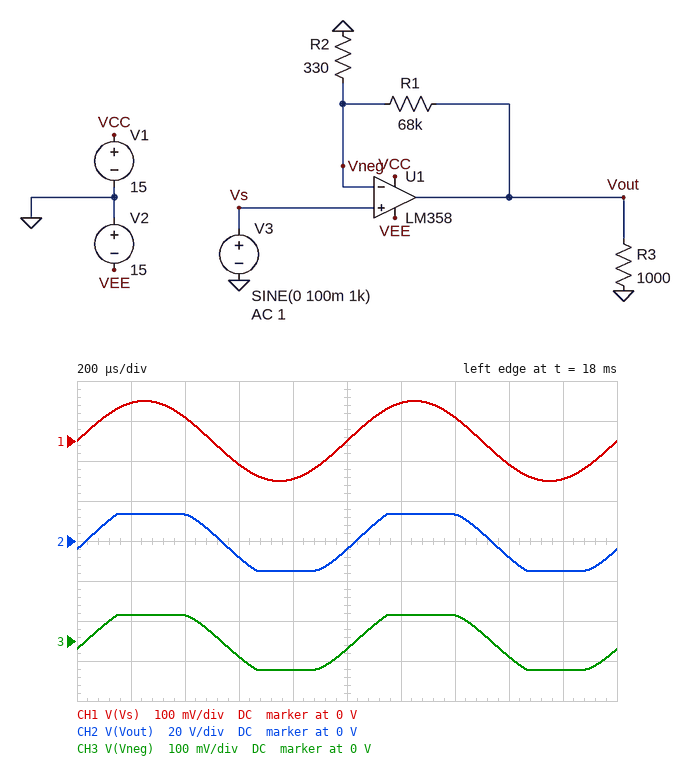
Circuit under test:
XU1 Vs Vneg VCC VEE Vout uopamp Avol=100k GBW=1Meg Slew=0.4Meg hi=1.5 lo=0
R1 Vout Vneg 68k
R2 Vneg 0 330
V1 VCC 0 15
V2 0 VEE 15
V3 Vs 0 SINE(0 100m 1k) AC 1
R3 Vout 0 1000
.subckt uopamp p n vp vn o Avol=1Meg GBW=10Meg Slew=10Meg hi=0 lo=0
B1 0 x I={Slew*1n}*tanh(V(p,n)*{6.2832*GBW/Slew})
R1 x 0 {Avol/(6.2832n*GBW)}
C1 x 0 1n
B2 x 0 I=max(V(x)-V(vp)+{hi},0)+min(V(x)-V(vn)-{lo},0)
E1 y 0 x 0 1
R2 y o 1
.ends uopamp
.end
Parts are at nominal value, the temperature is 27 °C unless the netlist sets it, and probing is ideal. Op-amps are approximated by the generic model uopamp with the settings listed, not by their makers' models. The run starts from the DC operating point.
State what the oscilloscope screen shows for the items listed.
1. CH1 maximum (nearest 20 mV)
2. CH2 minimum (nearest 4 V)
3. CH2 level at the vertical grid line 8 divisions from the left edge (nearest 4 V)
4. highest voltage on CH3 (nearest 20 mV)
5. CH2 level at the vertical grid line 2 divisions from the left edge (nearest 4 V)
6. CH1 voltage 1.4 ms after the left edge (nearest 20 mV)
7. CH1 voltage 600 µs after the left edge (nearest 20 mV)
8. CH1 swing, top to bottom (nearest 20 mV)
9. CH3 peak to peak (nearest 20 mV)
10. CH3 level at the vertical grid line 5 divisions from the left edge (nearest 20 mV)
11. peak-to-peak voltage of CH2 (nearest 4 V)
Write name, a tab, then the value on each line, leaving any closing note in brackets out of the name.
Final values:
CH1 maximum	100 mV
CH2 minimum	-16 V
CH2 level at the vertical grid line 8 divisions from the left edge	-8 V
highest voltage on CH3	60 mV
CH2 level at the vertical grid line 2 divisions from the left edge	12 V
CH1 voltage 1.4 ms after the left edge	60 mV
CH1 voltage 600 µs after the left edge	-60 mV
CH1 swing, top to bottom	200 mV
CH3 peak to peak	140 mV
CH3 level at the vertical grid line 5 divisions from the left edge	-20 mV
peak-to-peak voltage of CH2	28 V
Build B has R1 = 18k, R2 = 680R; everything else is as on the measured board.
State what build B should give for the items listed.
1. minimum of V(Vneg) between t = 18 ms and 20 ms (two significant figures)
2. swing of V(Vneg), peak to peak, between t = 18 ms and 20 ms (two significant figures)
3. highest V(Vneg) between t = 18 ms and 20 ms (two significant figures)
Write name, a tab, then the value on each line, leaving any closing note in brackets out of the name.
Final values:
minimum of V(Vneg) between t = 18 ms and 20 ms	-100 mV
swing of V(Vneg), peak to peak, between t = 18 ms and 20 ms	200 mV
highest V(Vneg) between t = 18 ms and 20 ms	100 mV
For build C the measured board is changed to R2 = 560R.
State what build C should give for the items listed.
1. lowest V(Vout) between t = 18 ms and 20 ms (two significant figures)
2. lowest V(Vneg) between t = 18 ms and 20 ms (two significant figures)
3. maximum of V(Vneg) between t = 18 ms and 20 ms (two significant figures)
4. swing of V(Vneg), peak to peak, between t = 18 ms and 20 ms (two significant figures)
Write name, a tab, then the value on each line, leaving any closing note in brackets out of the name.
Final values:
lowest V(Vout) between t = 18 ms and 20 ms	-12 V
lowest V(Vneg) between t = 18 ms and 20 ms	-99 mV
maximum of V(Vneg) between t = 18 ms and 20 ms	99 mV
swing of V(Vneg), peak to peak, between t = 18 ms and 20 ms	200 mV
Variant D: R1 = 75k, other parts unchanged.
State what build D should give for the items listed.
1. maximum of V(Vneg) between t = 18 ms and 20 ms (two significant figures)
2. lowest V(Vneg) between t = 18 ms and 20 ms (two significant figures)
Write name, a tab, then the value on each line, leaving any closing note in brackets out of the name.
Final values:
maximum of V(Vneg) between t = 18 ms and 20 ms	59 mV
lowest V(Vneg) between t = 18 ms and 20 ms	-66 mV
